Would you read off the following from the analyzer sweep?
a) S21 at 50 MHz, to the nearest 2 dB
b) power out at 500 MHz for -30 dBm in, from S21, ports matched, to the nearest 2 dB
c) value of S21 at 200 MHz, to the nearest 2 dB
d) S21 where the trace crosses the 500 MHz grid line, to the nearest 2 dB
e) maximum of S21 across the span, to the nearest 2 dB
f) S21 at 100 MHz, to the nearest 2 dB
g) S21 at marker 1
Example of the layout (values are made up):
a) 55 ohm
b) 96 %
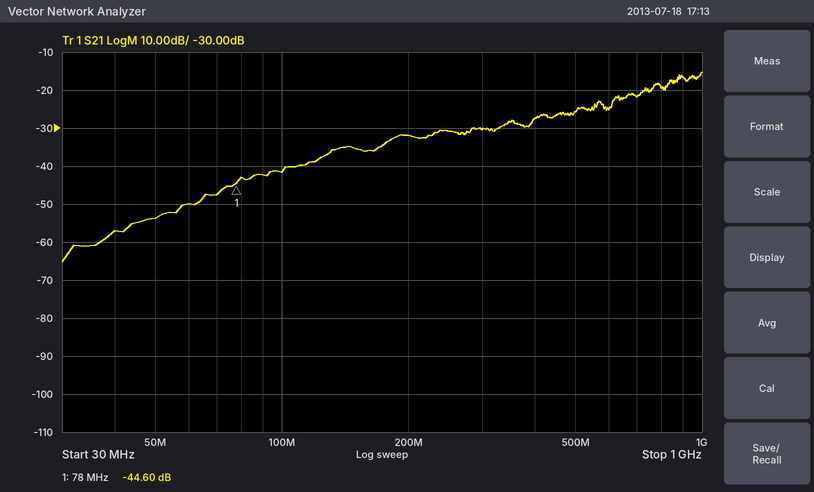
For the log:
a) -54 dB
b) -56 dBm
c) -32 dB
d) -26 dB
e) -16 dB
f) -42 dB
g) -44.60 dB
